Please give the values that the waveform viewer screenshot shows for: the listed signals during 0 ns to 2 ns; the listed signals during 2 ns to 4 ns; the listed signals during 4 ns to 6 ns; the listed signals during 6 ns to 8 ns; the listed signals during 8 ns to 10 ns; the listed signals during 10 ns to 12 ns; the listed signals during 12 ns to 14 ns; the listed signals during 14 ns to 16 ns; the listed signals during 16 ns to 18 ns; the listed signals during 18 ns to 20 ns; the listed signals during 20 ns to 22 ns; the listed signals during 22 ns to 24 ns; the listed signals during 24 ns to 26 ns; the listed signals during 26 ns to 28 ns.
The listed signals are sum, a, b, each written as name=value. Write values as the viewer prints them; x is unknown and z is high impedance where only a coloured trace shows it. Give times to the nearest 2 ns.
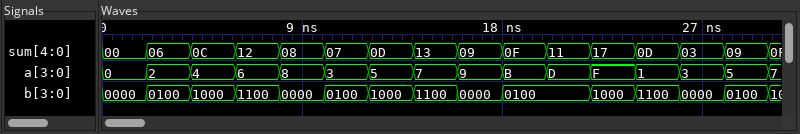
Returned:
sum=00, a=0, b=0000
sum=06, a=2, b=0100
sum=0C, a=4, b=1000
sum=12, a=6, b=1100
sum=08, a=8, b=0000
sum=07, a=3, b=0100
sum=0D, a=5, b=1000
sum=13, a=7, b=1100
sum=09, a=9, b=0000
sum=0F, a=B, b=0100
sum=11, a=D, b=0100
sum=17, a=F, b=1000
sum=0D, a=1, b=1100
sum=03, a=3, b=0000
